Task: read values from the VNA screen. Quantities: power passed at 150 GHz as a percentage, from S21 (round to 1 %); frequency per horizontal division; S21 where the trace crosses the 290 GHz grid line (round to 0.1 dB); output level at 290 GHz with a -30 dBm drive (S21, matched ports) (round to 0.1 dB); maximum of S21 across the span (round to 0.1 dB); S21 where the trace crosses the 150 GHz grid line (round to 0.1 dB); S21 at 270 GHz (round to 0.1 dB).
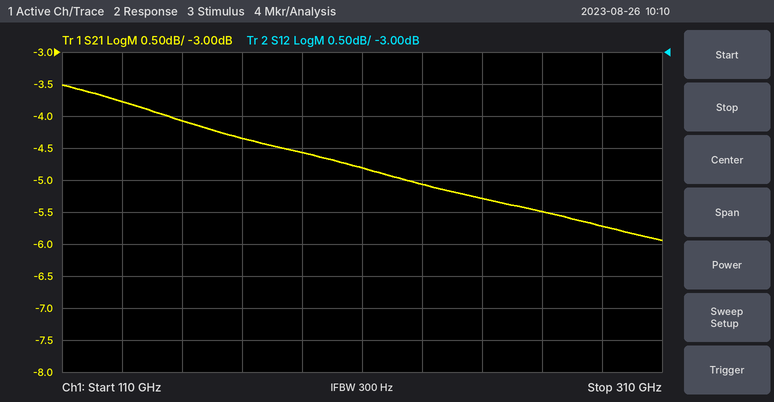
39 %
20 GHz
-5.7 dB
-35.7 dBm
-3.5 dB
-4.1 dB
-5.5 dB
